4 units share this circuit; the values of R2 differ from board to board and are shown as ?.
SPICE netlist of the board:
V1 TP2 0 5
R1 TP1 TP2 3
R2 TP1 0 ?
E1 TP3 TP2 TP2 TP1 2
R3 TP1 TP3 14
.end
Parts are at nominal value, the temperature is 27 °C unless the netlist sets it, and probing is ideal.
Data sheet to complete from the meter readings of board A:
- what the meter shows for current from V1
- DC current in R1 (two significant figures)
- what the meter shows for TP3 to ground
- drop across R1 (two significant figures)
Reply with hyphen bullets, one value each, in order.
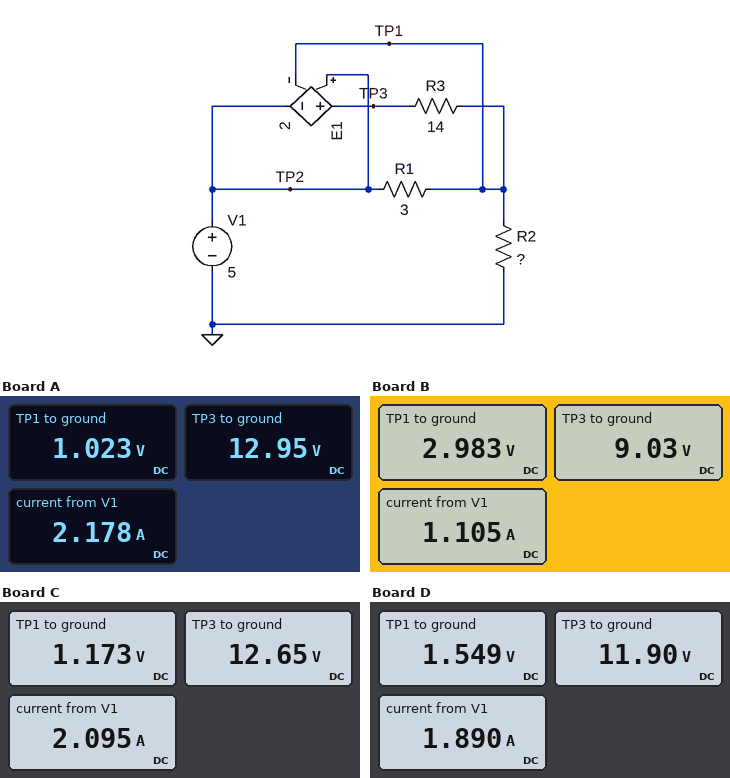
- 2.178 A
- 1.3 A
- 12.95 V
- 4.0 V
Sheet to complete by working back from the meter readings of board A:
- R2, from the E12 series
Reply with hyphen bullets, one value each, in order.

- 0.47 Ω
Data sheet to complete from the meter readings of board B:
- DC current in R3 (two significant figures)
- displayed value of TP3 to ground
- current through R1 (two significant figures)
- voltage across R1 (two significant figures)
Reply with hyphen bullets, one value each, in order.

- 430 mA
- 9.03 V
- 670 mA
- 2.0 V
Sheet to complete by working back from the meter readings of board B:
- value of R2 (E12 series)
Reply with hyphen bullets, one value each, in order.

- 2.7 Ω
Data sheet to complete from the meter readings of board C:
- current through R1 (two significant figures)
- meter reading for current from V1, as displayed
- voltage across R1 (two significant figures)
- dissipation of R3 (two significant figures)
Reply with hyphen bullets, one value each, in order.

- 1.3 A
- 2.095 A
- 3.8 V
- 9.4 W
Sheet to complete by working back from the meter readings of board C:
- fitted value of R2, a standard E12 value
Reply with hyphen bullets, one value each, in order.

- 0.56 Ω
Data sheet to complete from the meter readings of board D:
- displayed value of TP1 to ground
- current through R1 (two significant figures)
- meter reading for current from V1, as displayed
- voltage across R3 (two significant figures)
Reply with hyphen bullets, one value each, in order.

- 1.549 V
- 1.2 A
- 1.890 A
- 10 V
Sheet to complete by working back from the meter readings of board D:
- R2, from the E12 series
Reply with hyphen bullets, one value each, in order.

- 0.82 Ω
